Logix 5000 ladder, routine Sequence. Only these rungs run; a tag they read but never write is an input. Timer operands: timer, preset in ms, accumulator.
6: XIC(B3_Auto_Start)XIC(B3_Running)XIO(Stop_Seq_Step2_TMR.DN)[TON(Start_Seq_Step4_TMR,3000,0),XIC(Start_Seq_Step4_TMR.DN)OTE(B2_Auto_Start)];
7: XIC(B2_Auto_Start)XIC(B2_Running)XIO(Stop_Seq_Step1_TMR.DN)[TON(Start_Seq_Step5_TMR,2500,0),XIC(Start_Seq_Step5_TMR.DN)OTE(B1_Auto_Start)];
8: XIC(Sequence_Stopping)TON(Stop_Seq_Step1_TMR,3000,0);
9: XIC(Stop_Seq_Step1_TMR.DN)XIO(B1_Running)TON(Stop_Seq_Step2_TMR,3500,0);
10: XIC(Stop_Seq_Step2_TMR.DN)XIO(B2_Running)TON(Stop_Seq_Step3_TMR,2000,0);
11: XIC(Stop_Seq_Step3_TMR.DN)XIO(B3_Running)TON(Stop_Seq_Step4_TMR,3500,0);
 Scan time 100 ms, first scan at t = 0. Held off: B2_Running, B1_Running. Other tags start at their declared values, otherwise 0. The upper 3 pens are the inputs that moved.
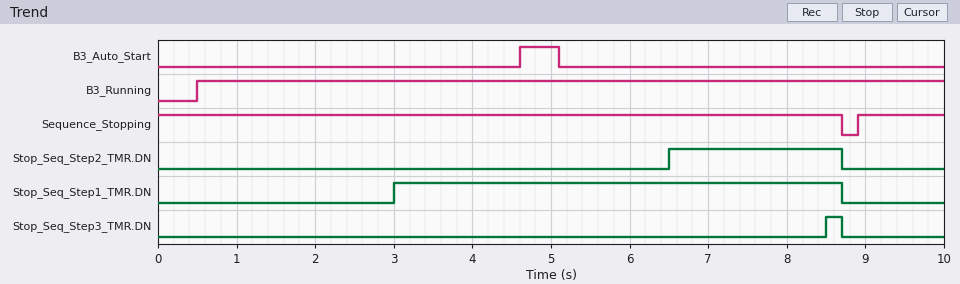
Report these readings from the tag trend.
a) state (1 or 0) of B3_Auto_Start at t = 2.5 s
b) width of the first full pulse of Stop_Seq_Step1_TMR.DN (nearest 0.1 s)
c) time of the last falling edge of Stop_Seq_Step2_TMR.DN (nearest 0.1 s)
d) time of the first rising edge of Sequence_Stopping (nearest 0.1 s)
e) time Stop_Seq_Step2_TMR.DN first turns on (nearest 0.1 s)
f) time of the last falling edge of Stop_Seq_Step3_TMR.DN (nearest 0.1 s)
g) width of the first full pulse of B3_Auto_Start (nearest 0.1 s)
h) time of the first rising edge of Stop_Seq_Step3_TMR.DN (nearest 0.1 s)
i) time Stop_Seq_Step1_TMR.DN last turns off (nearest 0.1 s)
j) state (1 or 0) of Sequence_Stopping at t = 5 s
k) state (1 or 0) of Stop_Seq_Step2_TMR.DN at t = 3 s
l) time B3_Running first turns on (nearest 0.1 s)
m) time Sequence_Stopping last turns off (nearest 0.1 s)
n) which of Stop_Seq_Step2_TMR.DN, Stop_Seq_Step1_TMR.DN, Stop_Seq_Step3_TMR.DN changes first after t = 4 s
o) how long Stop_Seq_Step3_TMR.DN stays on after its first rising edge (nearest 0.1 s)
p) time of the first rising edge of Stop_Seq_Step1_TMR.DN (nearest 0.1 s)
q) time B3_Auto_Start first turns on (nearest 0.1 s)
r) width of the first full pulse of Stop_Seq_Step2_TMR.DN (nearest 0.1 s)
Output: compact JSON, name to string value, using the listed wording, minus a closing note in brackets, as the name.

{"state (1 or 0) of B3_Auto_Start at t = 2.5 s": "0", "width of the first full pulse of Stop_Seq_Step1_TMR.DN": "5.7 s", "time of the last falling edge of Stop_Seq_Step2_TMR.DN": "8.7 s", "time of the first rising edge of Sequence_Stopping": "8.9 s", "time Stop_Seq_Step2_TMR.DN first turns on": "6.5 s", "time of the last falling edge of Stop_Seq_Step3_TMR.DN": "8.7 s", "width of the first full pulse of B3_Auto_Start": "0.5 s", "time of the first rising edge of Stop_Seq_Step3_TMR.DN": "8.5 s", "time Stop_Seq_Step1_TMR.DN last turns off": "8.7 s", "state (1 or 0) of Sequence_Stopping at t = 5 s": "1", "state (1 or 0) of Stop_Seq_Step2_TMR.DN at t = 3 s": "0", "time B3_Running first turns on": "0.5 s", "time Sequence_Stopping last turns off": "8.7 s", "which of Stop_Seq_Step2_TMR.DN, Stop_Seq_Step1_TMR.DN, Stop_Seq_Step3_TMR.DN changes first after t = 4 s": "Stop_Seq_Step2_TMR.DN", "how long Stop_Seq_Step3_TMR.DN stays on after its first rising edge": "0.2 s", "time of the first rising edge of Stop_Seq_Step1_TMR.DN": "3.0 s", "time B3_Auto_Start first turns on": "4.6 s", "width of the first full pulse of Stop_Seq_Step2_TMR.DN": "2.2 s"}
